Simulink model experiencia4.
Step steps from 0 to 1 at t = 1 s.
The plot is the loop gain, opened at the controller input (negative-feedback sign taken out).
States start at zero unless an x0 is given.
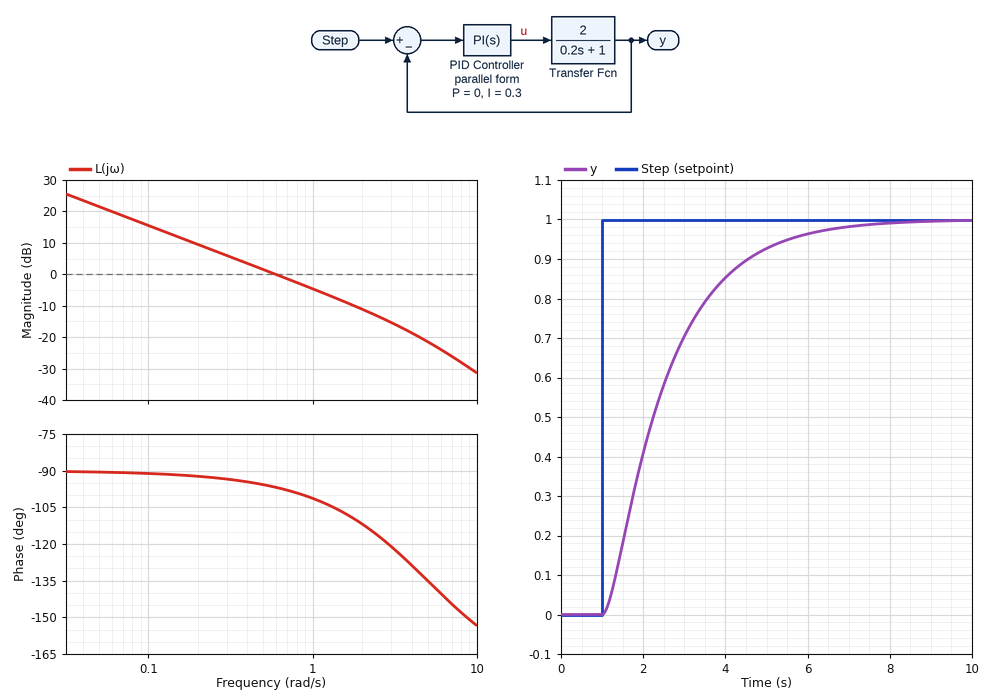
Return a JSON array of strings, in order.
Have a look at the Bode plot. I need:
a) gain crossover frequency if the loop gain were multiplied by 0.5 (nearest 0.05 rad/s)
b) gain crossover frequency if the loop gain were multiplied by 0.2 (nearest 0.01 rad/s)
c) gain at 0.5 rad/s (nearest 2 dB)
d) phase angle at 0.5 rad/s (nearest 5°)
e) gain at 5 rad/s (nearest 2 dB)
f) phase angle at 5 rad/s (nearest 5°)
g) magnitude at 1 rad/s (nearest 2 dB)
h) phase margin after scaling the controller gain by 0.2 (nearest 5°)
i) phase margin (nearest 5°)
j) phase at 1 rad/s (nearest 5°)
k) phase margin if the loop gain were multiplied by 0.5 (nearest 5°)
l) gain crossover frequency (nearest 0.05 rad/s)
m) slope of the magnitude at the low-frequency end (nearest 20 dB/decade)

["0.30 rad/s", "0.12 rad/s", "2 dB", "-95°", "-22 dB", "-135°", "-4 dB", "90°", "85°", "-100°", "85°", "0.60 rad/s", "-20 dB/decade"]
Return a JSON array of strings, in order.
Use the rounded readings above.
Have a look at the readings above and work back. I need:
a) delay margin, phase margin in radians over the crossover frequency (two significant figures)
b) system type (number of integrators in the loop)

["2.5 s", "1"]
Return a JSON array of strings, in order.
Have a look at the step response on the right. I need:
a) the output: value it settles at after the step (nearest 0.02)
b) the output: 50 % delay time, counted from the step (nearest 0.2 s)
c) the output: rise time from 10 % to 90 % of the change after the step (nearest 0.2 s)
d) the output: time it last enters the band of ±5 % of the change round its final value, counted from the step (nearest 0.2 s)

["1.00", "1.2 s", "3.2 s", "4.6 s"]
